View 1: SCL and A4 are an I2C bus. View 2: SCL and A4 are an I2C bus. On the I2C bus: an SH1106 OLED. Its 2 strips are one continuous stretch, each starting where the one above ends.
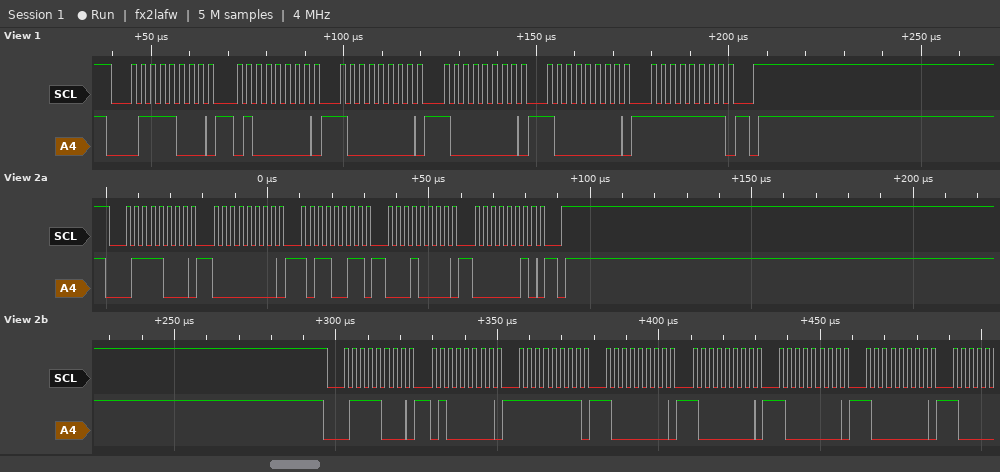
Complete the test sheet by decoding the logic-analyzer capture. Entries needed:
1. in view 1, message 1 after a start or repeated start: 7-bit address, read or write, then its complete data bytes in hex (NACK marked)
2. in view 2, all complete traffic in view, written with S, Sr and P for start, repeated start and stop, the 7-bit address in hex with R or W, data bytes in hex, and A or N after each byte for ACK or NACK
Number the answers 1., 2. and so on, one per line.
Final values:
1. 0x3C write: 40 80 80 80 FF
2. S 3CW A 00 A B3 A 10 A 02 A P S 3CW A 40 A FF A 80 A 80 A 80 A 80 A
